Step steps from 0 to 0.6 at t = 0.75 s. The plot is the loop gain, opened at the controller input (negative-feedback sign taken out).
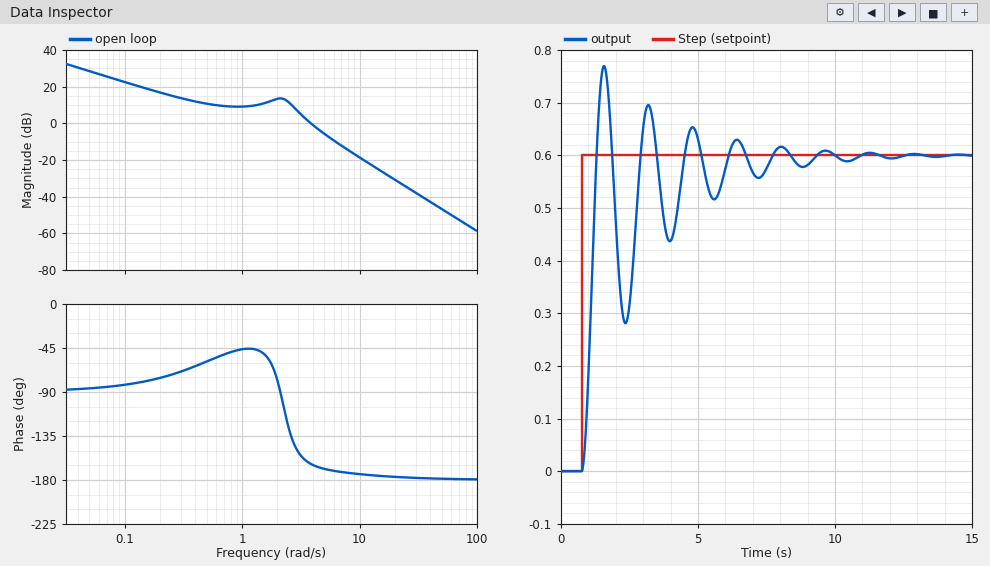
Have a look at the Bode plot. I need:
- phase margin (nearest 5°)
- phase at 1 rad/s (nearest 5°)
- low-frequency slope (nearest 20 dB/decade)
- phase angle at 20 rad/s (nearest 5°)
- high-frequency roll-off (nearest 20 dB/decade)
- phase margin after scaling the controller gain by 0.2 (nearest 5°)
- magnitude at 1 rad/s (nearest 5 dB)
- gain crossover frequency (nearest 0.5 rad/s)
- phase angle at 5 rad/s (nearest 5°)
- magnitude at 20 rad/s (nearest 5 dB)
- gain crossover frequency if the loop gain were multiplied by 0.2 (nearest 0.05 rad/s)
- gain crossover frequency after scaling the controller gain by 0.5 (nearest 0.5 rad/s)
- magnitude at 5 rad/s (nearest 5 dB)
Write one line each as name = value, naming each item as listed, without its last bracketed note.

phase margin = 15°
phase at 1 rad/s = -45°
low-frequency slope = -20 dB/decade
phase angle at 20 rad/s = -175°
high-frequency roll-off = -40 dB/decade
phase margin after scaling the controller gain by 0.2 = 110°
magnitude at 1 rad/s = 10 dB
gain crossover frequency = 4.0 rad/s
phase angle at 5 rad/s = -170°
magnitude at 20 rad/s = -30 dB
gain crossover frequency if the loop gain were multiplied by 0.2 = 0.30 rad/s
gain crossover frequency after scaling the controller gain by 0.5 = 3.0 rad/s
magnitude at 5 rad/s = -5 dB
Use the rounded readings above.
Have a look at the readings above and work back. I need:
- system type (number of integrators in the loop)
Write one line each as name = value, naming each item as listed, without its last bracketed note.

system type = 1
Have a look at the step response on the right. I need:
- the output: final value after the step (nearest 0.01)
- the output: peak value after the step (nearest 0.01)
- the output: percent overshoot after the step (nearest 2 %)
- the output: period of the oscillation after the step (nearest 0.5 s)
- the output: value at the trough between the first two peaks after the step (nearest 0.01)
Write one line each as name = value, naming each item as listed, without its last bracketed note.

the output: final value after the step = 0.60
the output: peak value after the step = 0.77
the output: percent overshoot after the step = 28 %
the output: period of the oscillation after the step = 1.5 s
the output: value at the trough between the first two peaks after the step = 0.28
